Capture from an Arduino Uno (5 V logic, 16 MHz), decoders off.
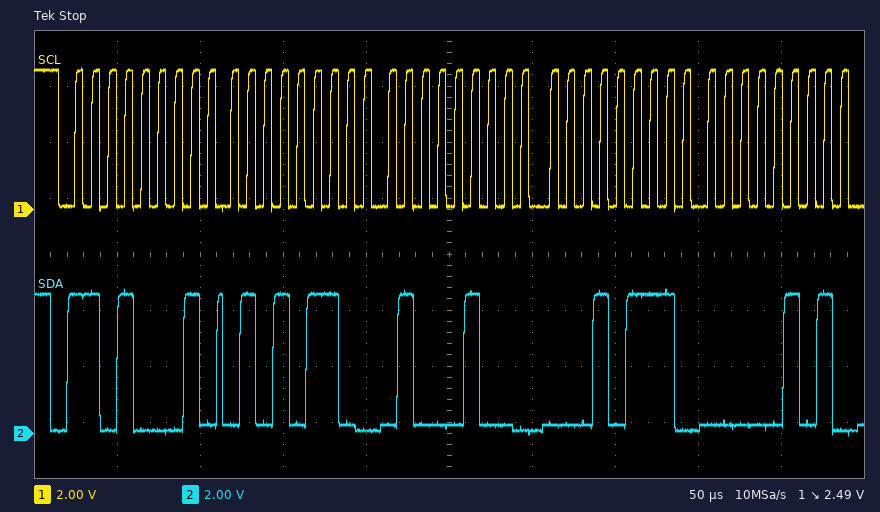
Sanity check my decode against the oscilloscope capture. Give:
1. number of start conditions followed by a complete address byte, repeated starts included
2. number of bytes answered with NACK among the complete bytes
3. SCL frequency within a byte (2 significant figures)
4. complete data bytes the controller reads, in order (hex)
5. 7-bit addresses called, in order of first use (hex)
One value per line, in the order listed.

1
0
100 kHz
56 44 17 05
0x68
